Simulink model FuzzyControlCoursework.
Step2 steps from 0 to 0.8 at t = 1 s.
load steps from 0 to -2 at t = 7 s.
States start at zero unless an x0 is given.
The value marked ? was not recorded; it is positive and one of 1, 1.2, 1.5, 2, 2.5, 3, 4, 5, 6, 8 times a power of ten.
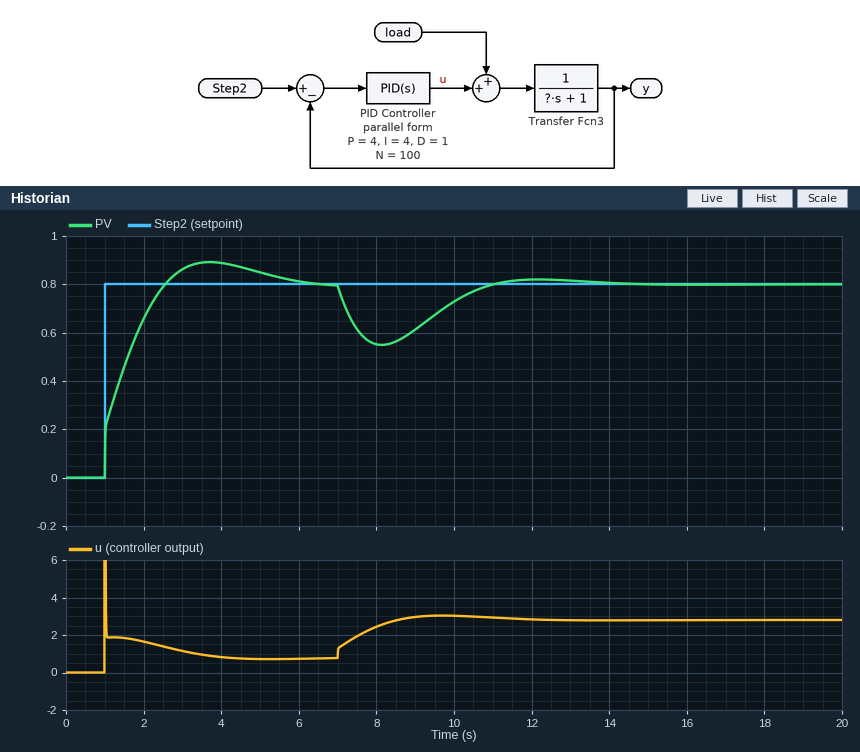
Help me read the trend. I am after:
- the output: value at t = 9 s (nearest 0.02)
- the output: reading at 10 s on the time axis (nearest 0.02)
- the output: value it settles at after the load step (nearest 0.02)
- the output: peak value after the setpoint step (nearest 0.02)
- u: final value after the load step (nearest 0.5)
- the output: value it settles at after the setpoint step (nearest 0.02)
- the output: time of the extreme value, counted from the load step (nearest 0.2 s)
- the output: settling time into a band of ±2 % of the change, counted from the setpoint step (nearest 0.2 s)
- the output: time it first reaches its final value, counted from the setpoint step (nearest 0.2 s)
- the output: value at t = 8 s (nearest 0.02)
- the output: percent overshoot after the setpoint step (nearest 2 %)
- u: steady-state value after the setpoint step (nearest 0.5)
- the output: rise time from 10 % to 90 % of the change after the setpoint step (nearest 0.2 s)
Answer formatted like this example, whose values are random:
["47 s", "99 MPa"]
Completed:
["0.62", "0.72", "0.80", "0.90", "3.0", "0.80", "1.2 s", "4.8 s", "1.6 s", "0.56", "12 %", "1.0", "1.2 s"]
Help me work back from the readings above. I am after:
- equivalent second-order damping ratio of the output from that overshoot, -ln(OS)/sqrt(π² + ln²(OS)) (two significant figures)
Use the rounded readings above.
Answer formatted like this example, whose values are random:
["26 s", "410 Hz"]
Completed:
["0.56"]
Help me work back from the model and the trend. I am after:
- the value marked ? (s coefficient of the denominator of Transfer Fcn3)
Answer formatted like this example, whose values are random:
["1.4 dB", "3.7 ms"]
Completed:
["3"]
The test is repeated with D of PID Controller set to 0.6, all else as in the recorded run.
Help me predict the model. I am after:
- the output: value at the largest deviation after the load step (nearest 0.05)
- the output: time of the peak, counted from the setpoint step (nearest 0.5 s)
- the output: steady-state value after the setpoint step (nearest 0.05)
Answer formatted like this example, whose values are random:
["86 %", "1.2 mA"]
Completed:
["0.55", "2.5 s", "0.80"]
